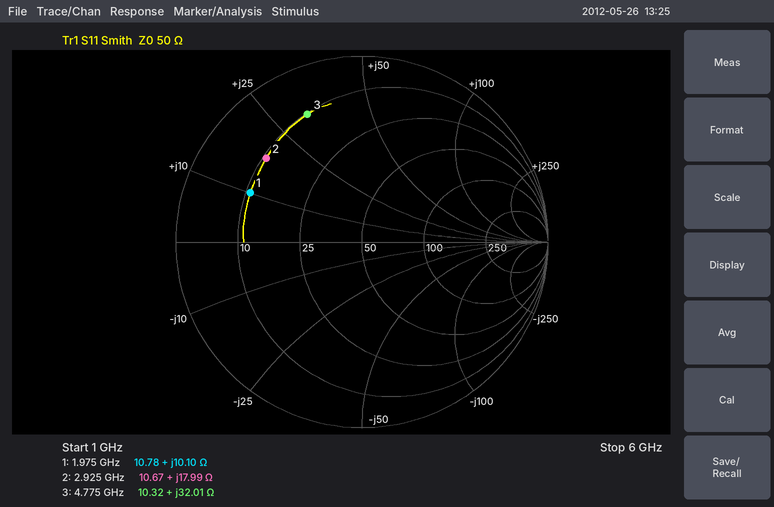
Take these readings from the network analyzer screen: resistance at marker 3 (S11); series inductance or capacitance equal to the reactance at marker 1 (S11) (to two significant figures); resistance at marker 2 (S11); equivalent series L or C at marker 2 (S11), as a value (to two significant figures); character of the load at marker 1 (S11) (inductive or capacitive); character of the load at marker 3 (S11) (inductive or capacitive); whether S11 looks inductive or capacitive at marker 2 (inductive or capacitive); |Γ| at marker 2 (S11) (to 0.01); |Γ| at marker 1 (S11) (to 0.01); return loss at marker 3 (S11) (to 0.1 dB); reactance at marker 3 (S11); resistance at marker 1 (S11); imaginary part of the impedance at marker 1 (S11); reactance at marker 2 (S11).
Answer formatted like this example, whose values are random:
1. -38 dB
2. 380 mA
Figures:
1. 10.32 Ω
2. 810 pH
3. 10.67 Ω
4. 980 pH
5. inductive
6. inductive
7. inductive
8. 0.68
9. 0.66
10. 2.5 dB
11. +32.01 Ω
12. 10.78 Ω
13. +10.10 Ω
14. +17.99 Ω
